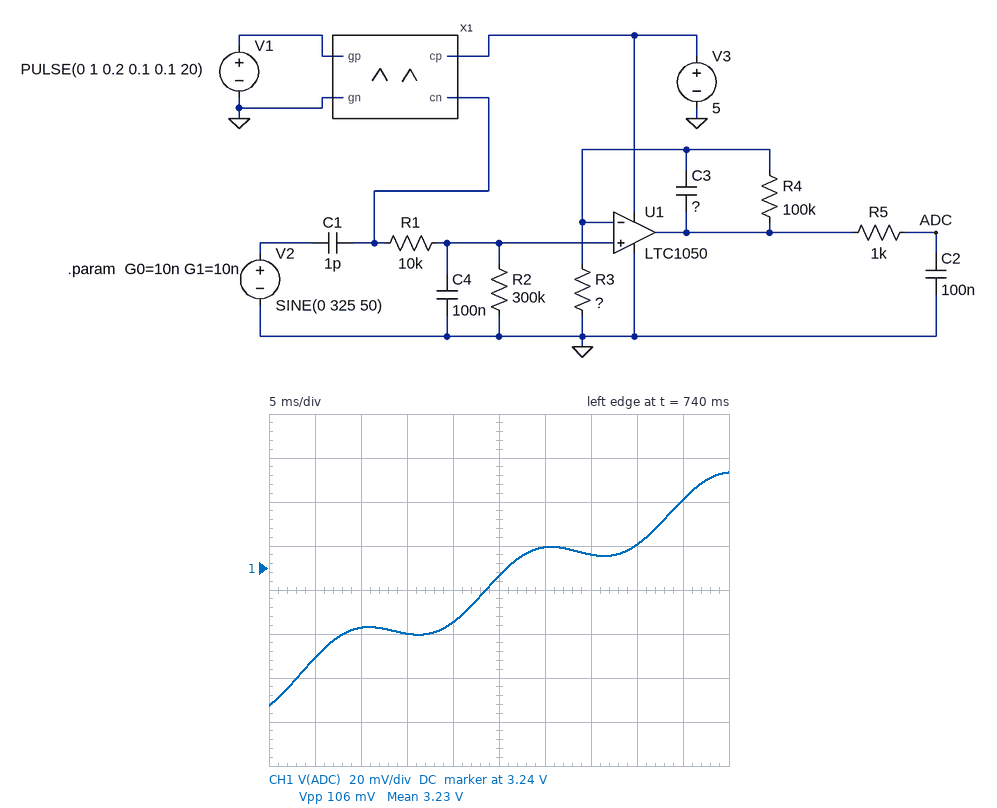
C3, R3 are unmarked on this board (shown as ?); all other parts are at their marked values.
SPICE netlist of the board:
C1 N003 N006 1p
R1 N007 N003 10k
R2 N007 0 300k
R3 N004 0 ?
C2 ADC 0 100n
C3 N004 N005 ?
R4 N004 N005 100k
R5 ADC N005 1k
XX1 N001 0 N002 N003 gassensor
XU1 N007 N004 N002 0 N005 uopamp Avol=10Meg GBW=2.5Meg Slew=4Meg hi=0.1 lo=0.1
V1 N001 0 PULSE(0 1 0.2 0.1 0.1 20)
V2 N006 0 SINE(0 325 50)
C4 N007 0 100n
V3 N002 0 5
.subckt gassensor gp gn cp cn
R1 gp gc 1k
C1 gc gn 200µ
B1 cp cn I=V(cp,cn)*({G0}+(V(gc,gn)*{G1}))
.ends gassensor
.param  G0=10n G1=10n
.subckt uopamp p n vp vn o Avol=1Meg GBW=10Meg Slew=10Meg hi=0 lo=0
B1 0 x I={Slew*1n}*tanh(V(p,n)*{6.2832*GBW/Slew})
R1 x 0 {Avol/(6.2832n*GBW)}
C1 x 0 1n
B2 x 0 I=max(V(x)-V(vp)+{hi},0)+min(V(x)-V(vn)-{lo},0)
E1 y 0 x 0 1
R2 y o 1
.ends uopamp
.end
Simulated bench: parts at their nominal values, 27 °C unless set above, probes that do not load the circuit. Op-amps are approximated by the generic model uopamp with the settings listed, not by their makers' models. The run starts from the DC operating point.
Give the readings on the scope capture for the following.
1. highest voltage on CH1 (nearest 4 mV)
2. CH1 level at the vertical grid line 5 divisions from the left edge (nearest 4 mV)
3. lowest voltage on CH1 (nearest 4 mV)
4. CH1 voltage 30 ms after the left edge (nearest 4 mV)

3.284 V
3.236 V
3.176 V
3.248 V
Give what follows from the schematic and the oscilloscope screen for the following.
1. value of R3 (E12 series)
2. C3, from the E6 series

820 Ω
1.5 µF
